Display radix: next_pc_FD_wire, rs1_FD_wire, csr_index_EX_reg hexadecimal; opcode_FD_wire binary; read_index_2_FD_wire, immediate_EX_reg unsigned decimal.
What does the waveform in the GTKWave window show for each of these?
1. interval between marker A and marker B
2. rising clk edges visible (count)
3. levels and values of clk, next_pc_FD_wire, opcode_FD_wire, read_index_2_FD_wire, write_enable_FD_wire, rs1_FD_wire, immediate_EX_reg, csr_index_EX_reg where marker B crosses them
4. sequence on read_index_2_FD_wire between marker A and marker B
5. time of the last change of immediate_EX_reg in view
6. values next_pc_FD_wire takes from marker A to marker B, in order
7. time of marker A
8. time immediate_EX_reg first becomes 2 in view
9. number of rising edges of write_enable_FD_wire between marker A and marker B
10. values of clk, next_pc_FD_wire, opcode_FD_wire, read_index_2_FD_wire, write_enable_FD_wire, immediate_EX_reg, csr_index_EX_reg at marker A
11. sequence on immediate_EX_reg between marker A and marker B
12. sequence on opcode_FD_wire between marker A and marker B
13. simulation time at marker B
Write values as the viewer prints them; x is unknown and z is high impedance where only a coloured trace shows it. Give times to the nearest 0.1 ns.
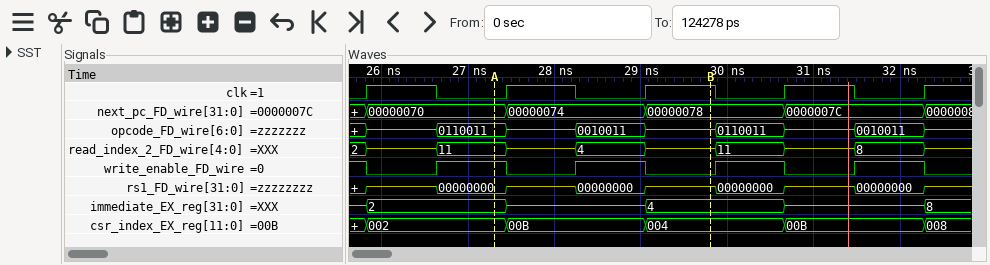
2.5 ns
5
clk=1, next_pc_FD_wire=00000078, opcode_FD_wire=z, read_index_2_FD_wire=z, write_enable_FD_wire=0, rs1_FD_wire=z, immediate_EX_reg=4, csr_index_EX_reg=004
11, z, 4, z
32.3 ns
00000070, 00000074, 00000078
27.3 ns
25.8 ns
1
clk=0, next_pc_FD_wire=00000070, opcode_FD_wire=0110011, read_index_2_FD_wire=11, write_enable_FD_wire=1, immediate_EX_reg=2, csr_index_EX_reg=002
2, z, 4
0110011, z, 0010011, z
29.8 ns
